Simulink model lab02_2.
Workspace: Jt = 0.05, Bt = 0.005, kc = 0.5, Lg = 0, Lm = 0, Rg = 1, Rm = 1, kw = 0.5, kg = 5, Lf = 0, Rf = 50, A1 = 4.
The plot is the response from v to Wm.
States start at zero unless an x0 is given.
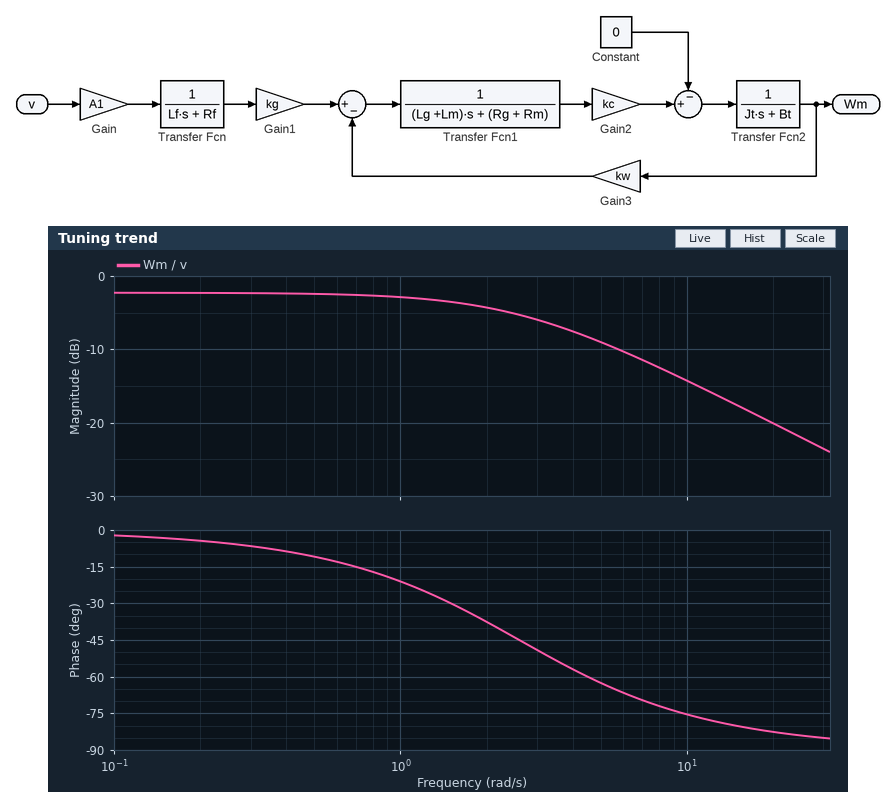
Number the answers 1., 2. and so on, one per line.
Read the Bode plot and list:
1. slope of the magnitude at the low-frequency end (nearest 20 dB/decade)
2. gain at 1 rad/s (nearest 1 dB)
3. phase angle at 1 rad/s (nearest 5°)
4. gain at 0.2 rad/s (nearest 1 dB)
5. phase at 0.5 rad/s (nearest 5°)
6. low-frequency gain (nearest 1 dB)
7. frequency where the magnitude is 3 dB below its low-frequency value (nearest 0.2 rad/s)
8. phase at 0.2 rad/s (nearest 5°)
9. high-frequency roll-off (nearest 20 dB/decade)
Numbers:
1. 0 dB/decade
2. -3 dB
3. -20°
4. -2 dB
5. -10°
6. -2 dB
7. 2.6 rad/s
8. -5°
9. -20 dB/decade
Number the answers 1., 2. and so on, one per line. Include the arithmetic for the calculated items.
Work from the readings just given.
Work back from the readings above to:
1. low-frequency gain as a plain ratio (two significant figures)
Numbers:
1. 10^(-2 / 20) = 0.79
